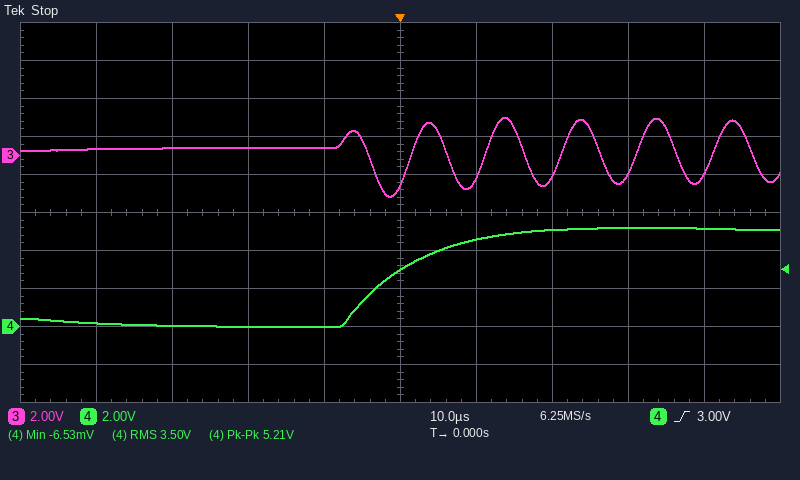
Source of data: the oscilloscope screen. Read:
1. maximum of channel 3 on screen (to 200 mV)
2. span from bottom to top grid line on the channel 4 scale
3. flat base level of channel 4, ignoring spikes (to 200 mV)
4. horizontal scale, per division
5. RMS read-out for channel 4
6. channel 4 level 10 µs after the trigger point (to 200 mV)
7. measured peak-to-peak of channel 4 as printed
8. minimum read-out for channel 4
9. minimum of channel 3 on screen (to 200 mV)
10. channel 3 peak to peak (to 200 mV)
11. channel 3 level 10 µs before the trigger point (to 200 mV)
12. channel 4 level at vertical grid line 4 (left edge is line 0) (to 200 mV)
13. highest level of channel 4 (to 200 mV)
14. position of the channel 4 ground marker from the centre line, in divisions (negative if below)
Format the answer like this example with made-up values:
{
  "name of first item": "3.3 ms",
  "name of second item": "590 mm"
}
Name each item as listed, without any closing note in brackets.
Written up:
{
  "maximum of channel 3 on screen": "2.0 V",
  "span from bottom to top grid line on the channel 4 scale": "20 V",
  "flat base level of channel 4, ignoring spikes": "0.0 V",
  "horizontal scale, per division": "10 µs",
  "RMS read-out for channel 4": "3.50 V",
  "channel 4 level 10 µs after the trigger point": "4.6 V",
  "measured peak-to-peak of channel 4 as printed": "5.21 V",
  "minimum read-out for channel 4": "-6.53 mV",
  "minimum of channel 3 on screen": "-2.2 V",
  "channel 3 peak to peak": "4.2 V",
  "channel 3 level 10 µs before the trigger point": "400 mV",
  "channel 4 level at vertical grid line 4 (left edge is line 0)": "0.0 V",
  "highest level of channel 4": "5.2 V",
  "position of the channel 4 ground marker from the centre line, in divisions": "-3.0 div"
}
